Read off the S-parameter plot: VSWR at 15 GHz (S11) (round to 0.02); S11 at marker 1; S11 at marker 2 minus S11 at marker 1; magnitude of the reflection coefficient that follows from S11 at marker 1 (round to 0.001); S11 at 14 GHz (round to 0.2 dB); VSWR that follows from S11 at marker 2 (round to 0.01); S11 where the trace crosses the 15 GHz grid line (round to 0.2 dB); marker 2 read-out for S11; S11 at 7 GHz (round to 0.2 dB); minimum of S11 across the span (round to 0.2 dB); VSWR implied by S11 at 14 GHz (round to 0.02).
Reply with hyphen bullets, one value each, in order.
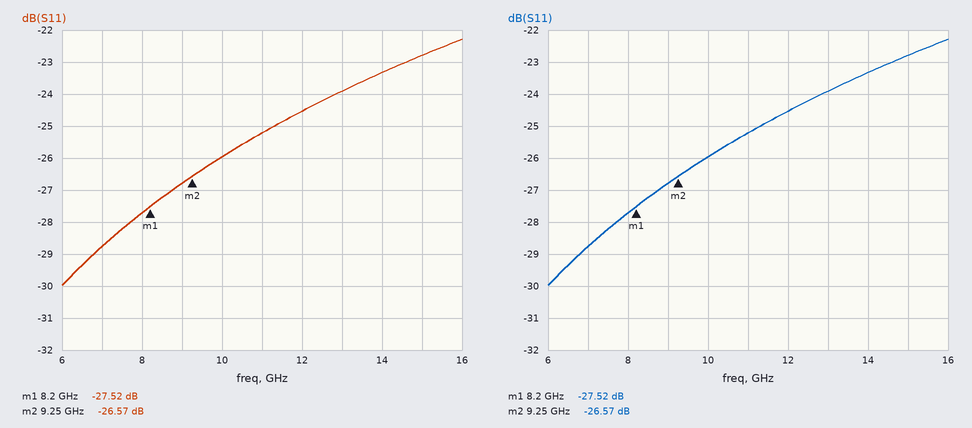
- 1.16
- -27.52 dB
- 0.95 dB
- 0.042
- -23.4 dB
- 1.10
- -22.8 dB
- -26.57 dB
- -28.8 dB
- -30.0 dB
- 1.14
